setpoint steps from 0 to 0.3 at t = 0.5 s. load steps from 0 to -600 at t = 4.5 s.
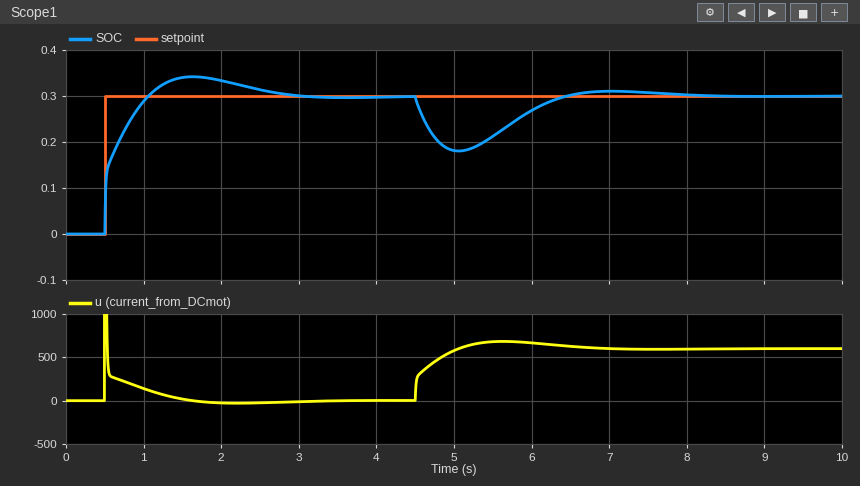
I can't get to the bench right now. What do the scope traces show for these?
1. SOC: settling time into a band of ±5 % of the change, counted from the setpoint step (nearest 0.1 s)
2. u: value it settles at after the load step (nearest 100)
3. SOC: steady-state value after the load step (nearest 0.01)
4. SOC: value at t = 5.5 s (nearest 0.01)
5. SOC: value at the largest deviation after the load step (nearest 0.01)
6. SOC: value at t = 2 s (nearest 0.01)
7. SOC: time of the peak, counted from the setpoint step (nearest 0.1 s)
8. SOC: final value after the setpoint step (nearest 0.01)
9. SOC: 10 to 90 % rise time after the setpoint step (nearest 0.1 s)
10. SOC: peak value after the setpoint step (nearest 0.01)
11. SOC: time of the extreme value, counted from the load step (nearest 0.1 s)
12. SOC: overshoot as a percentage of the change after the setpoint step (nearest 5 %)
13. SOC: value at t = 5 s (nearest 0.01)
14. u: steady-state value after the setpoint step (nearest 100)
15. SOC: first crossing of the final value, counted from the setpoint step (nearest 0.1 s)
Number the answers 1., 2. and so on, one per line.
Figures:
1. 2.0 s
2. 600
3. 0.30
4. 0.21
5. 0.18
6. 0.33
7. 1.1 s
8. 0.30
9. 0.4 s
10. 0.34
11. 0.6 s
12. 15 %
13. 0.18
14. 0
15. 0.6 s
